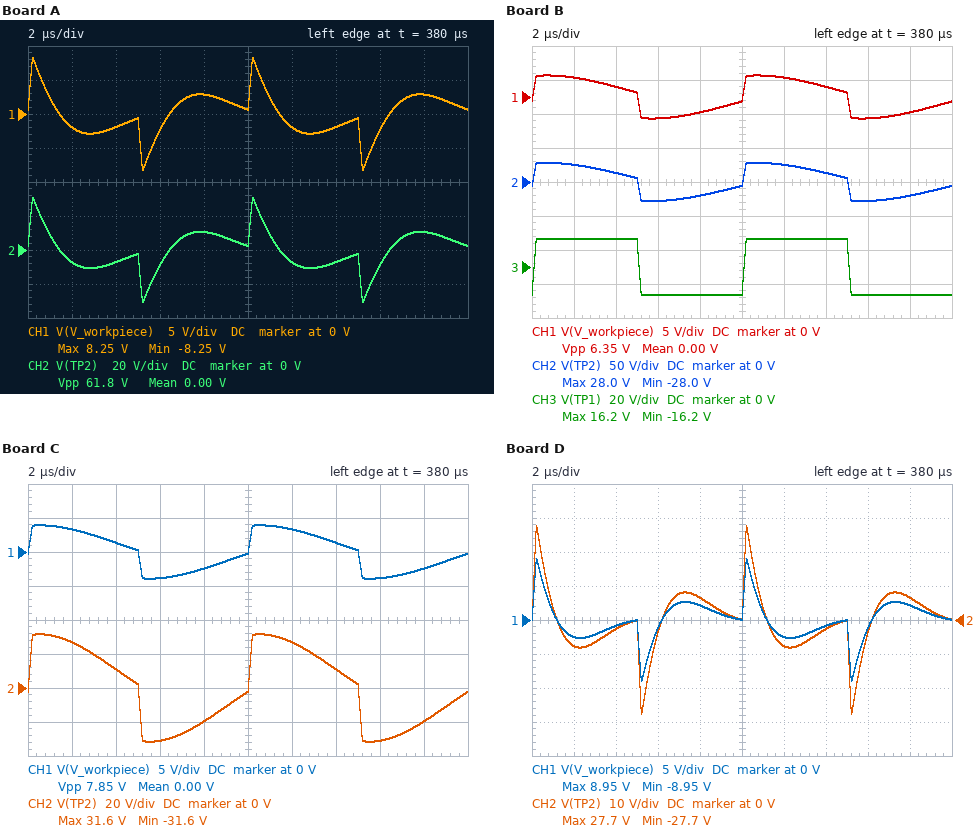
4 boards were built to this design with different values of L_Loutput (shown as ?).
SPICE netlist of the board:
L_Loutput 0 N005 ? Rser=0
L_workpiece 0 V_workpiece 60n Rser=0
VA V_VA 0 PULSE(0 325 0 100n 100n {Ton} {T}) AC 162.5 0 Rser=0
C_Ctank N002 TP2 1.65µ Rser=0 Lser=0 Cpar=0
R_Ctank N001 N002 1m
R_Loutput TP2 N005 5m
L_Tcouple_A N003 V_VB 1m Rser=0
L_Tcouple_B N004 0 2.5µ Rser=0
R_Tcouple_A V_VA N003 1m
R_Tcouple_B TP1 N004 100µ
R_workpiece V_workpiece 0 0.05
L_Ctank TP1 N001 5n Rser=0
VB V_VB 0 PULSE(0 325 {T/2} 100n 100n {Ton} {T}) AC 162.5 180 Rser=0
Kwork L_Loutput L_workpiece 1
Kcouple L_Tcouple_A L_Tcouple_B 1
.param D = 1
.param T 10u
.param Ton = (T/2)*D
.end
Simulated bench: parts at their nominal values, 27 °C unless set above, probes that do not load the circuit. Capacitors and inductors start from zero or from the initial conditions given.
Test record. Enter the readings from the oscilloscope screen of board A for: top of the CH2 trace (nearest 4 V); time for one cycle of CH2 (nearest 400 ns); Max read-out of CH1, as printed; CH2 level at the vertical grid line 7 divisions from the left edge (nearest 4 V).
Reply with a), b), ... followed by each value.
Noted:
a) 32 V
b) 10.0 µs
c) 8.25 V
d) -8 V
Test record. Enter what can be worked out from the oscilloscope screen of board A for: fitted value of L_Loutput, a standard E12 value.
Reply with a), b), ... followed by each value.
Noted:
a) 820 nH
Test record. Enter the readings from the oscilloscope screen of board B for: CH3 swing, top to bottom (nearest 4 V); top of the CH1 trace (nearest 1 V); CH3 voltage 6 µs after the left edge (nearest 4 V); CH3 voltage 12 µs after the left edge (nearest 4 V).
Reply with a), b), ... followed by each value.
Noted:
a) 32 V
b) 3 V
c) -16 V
d) 16 V
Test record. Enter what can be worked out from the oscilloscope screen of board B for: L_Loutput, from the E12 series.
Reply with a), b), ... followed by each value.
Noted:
a) 4.7 µH
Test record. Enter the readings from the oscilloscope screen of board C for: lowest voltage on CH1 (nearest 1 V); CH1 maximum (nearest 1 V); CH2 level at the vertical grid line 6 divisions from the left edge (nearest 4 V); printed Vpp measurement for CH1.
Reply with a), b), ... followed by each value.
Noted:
a) -4 V
b) 4 V
c) 28 V
d) 7.85 V
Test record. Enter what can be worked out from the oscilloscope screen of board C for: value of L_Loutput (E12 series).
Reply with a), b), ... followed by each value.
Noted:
a) 3.9 µH
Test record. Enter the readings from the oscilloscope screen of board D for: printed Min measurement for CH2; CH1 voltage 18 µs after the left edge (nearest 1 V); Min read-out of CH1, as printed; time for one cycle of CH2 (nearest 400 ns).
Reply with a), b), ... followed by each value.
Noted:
a) -27.7 V
b) 2 V
c) -8.95 V
d) 10.0 µs
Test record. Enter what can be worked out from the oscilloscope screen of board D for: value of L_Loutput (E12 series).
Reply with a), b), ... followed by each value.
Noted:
a) 560 nH
